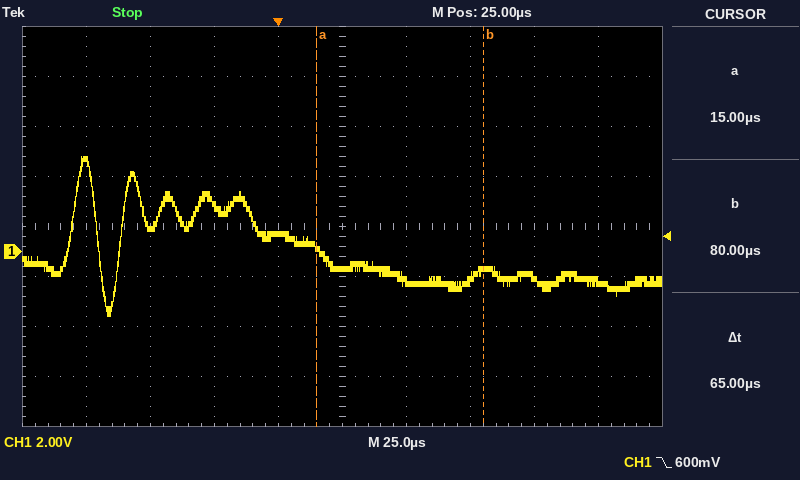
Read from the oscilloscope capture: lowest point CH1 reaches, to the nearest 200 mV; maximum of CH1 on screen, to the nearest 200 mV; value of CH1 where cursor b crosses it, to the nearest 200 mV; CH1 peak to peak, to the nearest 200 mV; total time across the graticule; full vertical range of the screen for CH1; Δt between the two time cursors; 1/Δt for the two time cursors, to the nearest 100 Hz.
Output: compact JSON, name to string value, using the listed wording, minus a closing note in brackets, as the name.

{"lowest point CH1 reaches, to the nearest 200 mV": "-2.6 V", "maximum of CH1 on screen, to the nearest 200 mV": "3.8 V", "value of CH1 where cursor b crosses it, to the nearest 200 mV": "-800 mV", "CH1 peak to peak, to the nearest 200 mV": "6.4 V", "total time across the graticule": "250 µs", "full vertical range of the screen for CH1": "16 V", "Δt between the two time cursors": "65 µs", "1/Δt for the two time cursors, to the nearest 100 Hz": "15.4 kHz"}
